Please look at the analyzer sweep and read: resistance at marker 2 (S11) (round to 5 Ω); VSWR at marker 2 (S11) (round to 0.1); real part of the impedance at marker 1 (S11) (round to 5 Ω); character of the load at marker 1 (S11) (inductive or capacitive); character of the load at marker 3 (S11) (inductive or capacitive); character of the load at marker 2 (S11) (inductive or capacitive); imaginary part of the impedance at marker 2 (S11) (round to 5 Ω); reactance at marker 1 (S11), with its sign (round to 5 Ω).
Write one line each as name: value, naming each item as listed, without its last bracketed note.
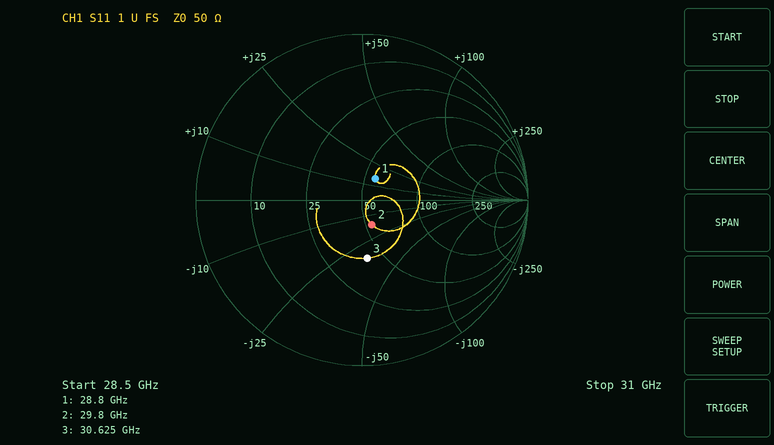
resistance at marker 2 (S11): 55 Ω
VSWR at marker 2 (S11): 1.4
real part of the impedance at marker 1 (S11): 55 Ω
character of the load at marker 1 (S11): inductive
character of the load at marker 3 (S11): capacitive
character of the load at marker 2 (S11): capacitive
imaginary part of the impedance at marker 2 (S11): -15 Ω
reactance at marker 1 (S11), with its sign: +15 Ω
